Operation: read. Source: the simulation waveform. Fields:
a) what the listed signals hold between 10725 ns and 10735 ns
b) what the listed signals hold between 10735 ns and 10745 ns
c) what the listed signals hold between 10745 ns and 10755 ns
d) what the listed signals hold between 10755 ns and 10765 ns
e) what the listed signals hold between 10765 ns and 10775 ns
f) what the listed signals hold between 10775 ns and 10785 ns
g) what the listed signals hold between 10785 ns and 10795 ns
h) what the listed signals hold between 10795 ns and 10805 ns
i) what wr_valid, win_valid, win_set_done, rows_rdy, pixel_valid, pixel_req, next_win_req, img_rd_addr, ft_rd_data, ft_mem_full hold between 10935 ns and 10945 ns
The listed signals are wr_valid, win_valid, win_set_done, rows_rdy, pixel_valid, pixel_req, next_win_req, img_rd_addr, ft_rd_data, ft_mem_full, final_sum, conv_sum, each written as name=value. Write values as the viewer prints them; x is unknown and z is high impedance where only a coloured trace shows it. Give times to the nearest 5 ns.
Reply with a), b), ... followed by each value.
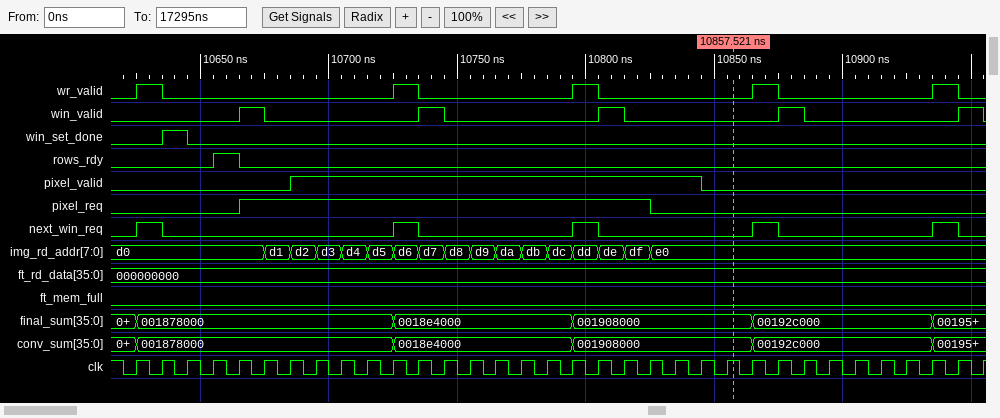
a) wr_valid=1, win_valid=0, win_set_done=0, rows_rdy=0, pixel_valid=1, pixel_req=1, next_win_req=1, img_rd_addr=d6, ft_rd_data=000000000, ft_mem_full=0, final_sum=0018e4000, conv_sum=0018e4000
b) wr_valid=0, win_valid=1, win_set_done=0, rows_rdy=0, pixel_valid=1, pixel_req=1, next_win_req=0, img_rd_addr=d7, ft_rd_data=000000000, ft_mem_full=0, final_sum=0018e4000, conv_sum=0018e4000
c) wr_valid=0, win_valid=0, win_set_done=0, rows_rdy=0, pixel_valid=1, pixel_req=1, next_win_req=0, img_rd_addr=d8, ft_rd_data=000000000, ft_mem_full=0, final_sum=0018e4000, conv_sum=0018e4000
d) wr_valid=0, win_valid=0, win_set_done=0, rows_rdy=0, pixel_valid=1, pixel_req=1, next_win_req=0, img_rd_addr=d9, ft_rd_data=000000000, ft_mem_full=0, final_sum=0018e4000, conv_sum=0018e4000
e) wr_valid=0, win_valid=0, win_set_done=0, rows_rdy=0, pixel_valid=1, pixel_req=1, next_win_req=0, img_rd_addr=da, ft_rd_data=000000000, ft_mem_full=0, final_sum=0018e4000, conv_sum=0018e4000
f) wr_valid=0, win_valid=0, win_set_done=0, rows_rdy=0, pixel_valid=1, pixel_req=1, next_win_req=0, img_rd_addr=db, ft_rd_data=000000000, ft_mem_full=0, final_sum=0018e4000, conv_sum=0018e4000
g) wr_valid=0, win_valid=0, win_set_done=0, rows_rdy=0, pixel_valid=1, pixel_req=1, next_win_req=0, img_rd_addr=dc, ft_rd_data=000000000, ft_mem_full=0, final_sum=0018e4000, conv_sum=0018e4000
h) wr_valid=1, win_valid=0, win_set_done=0, rows_rdy=0, pixel_valid=1, pixel_req=1, next_win_req=1, img_rd_addr=dd, ft_rd_data=000000000, ft_mem_full=0, final_sum=001908000, conv_sum=001908000
i) wr_valid=1, win_valid=0, win_set_done=0, rows_rdy=0, pixel_valid=0, pixel_req=0, next_win_req=1, img_rd_addr=e0, ft_rd_data=000000000, ft_mem_full=0
